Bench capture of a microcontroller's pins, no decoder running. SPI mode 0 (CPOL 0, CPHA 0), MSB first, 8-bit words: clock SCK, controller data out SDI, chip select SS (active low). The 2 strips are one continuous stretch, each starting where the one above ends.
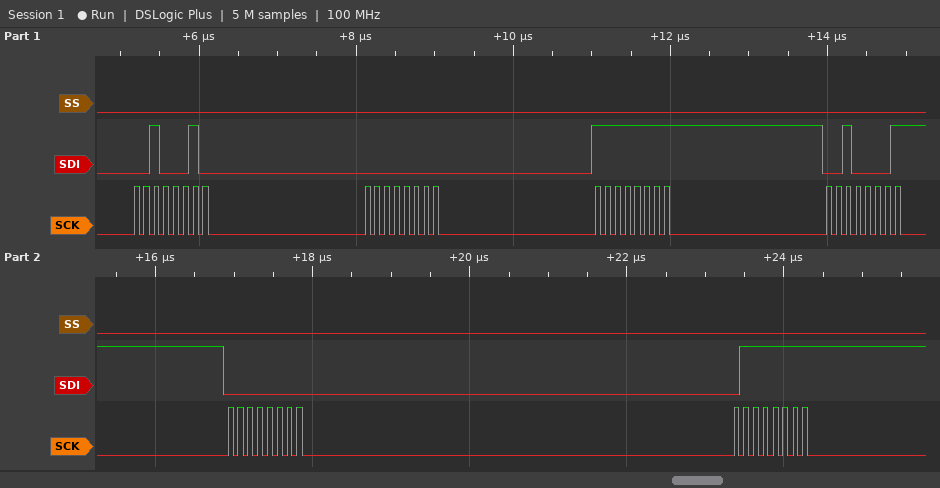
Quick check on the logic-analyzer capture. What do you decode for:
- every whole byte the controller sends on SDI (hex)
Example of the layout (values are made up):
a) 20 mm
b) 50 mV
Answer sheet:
a) 0x22 0x00 0xFF 0x21 0x00 0x7F
